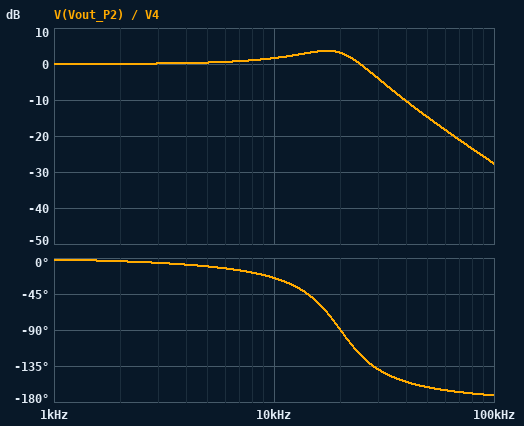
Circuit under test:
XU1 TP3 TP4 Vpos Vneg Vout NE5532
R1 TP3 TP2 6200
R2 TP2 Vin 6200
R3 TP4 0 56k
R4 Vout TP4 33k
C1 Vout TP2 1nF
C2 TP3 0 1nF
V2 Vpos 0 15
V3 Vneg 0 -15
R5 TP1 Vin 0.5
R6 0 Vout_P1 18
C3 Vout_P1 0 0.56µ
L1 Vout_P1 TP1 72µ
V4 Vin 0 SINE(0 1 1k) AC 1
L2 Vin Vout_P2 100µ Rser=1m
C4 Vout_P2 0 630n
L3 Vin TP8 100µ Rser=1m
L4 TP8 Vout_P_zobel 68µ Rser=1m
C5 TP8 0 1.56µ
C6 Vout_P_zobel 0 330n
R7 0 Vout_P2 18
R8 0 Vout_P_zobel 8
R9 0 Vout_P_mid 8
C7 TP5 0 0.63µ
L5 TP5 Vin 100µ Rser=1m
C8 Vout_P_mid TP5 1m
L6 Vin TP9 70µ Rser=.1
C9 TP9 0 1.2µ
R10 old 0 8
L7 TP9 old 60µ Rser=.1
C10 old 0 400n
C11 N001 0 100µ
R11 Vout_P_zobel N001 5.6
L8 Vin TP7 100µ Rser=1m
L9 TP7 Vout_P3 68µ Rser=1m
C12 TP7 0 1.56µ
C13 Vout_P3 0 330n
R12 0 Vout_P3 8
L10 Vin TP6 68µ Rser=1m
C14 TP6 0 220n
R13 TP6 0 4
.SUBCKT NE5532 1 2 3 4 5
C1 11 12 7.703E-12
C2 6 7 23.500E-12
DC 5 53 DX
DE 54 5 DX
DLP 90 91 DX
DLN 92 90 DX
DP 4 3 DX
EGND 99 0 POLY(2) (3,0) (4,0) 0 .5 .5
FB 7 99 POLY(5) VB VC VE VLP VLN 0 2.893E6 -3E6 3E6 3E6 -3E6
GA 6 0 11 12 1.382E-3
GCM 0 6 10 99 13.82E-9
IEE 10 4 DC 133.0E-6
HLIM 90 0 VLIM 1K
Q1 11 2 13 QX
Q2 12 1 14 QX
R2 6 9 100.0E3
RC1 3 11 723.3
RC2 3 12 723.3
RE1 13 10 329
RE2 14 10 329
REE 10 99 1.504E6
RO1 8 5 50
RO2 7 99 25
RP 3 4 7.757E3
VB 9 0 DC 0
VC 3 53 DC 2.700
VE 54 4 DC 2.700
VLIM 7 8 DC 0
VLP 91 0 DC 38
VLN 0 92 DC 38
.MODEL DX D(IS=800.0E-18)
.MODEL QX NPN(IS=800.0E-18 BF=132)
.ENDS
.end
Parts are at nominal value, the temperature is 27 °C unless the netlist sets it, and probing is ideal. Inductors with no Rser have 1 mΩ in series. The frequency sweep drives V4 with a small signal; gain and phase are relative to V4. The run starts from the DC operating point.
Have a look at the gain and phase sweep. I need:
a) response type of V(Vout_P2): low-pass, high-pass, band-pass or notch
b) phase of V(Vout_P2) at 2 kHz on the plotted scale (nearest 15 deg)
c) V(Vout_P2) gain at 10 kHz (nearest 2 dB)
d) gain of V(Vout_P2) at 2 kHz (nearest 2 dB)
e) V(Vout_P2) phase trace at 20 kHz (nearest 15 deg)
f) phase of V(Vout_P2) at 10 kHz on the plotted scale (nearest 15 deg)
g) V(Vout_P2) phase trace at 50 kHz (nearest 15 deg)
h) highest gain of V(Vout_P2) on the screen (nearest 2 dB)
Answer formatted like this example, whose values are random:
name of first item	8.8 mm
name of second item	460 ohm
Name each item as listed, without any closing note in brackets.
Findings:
response type of V(Vout_P2): low-pass, high-pass, band-pass or notch	low-pass
phase of V(Vout_P2) at 2 kHz on the plotted scale	0 deg
V(Vout_P2) gain at 10 kHz	2 dB
gain of V(Vout_P2) at 2 kHz	0 dB
V(Vout_P2) phase trace at 20 kHz	-90 deg
phase of V(Vout_P2) at 10 kHz on the plotted scale	-30 deg
V(Vout_P2) phase trace at 50 kHz	-165 deg
highest gain of V(Vout_P2) on the screen	4 dB
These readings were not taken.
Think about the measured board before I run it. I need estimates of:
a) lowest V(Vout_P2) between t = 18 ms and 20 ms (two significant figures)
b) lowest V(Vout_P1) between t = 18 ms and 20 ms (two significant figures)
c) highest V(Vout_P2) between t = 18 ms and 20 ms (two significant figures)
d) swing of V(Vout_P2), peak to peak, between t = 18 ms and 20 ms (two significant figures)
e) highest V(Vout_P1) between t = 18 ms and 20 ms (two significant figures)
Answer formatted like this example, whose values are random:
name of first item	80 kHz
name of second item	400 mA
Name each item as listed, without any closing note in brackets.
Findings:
lowest V(Vout_P2) between t = 18 ms and 20 ms	-1.0 V
lowest V(Vout_P1) between t = 18 ms and 20 ms	-970 mV
highest V(Vout_P2) between t = 18 ms and 20 ms	1.0 V
swing of V(Vout_P2), peak to peak, between t = 18 ms and 20 ms	2.0 V
highest V(Vout_P1) between t = 18 ms and 20 ms	970 mV
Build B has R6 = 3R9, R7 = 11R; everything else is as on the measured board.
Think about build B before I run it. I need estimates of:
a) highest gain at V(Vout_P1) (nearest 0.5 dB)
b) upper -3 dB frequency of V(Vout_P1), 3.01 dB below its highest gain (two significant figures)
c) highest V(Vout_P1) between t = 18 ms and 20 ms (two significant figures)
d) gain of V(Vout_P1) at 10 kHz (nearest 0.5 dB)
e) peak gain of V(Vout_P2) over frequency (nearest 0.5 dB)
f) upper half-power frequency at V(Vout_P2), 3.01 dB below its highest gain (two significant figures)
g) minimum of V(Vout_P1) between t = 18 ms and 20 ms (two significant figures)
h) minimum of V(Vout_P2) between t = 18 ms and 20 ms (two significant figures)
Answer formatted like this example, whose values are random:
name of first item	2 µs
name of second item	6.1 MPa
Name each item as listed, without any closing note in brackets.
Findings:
highest gain at V(Vout_P1)	-1.0 dB
upper -3 dB frequency of V(Vout_P1), 3.01 dB below its highest gain	11 kHz
highest V(Vout_P1) between t = 18 ms and 20 ms	880 mV
gain of V(Vout_P1) at 10 kHz	-3.5 dB
peak gain of V(Vout_P2) over frequency	0.5 dB
upper half-power frequency at V(Vout_P2), 3.01 dB below its highest gain	23 kHz
minimum of V(Vout_P1) between t = 18 ms and 20 ms	-880 mV
minimum of V(Vout_P2) between t = 18 ms and 20 ms	-1.0 V
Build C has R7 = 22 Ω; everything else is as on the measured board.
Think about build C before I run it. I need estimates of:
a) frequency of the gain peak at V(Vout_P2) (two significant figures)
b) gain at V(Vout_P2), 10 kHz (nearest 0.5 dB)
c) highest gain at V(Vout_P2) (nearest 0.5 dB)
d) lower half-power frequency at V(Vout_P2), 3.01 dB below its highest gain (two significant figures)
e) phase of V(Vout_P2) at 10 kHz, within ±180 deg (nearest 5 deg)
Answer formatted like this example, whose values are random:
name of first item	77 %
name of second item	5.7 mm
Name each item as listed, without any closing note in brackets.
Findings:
frequency of the gain peak at V(Vout_P2)	18 kHz
gain at V(Vout_P2), 10 kHz	2.0 dB
highest gain at V(Vout_P2)	5.0 dB
lower half-power frequency at V(Vout_P2), 3.01 dB below its highest gain	11 kHz
phase of V(Vout_P2) at 10 kHz, within ±180 deg	-20 deg
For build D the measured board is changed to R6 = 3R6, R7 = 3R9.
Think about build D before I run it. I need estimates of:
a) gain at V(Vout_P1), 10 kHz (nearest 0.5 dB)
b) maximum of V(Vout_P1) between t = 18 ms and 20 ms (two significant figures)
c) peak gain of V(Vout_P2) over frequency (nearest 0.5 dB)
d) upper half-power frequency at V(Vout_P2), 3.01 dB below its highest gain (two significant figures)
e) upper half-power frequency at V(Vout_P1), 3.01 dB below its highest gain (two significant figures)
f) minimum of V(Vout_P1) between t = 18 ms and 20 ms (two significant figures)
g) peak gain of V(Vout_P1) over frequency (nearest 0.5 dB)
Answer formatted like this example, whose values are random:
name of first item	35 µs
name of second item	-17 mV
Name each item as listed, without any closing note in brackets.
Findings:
gain at V(Vout_P1), 10 kHz	-4.0 dB
maximum of V(Vout_P1) between t = 18 ms and 20 ms	870 mV
peak gain of V(Vout_P2) over frequency	0 dB
upper half-power frequency at V(Vout_P2), 3.01 dB below its highest gain	6.9 kHz
upper half-power frequency at V(Vout_P1), 3.01 dB below its highest gain	10 kHz
minimum of V(Vout_P1) between t = 18 ms and 20 ms	-870 mV
peak gain of V(Vout_P1) over frequency	-1.0 dB
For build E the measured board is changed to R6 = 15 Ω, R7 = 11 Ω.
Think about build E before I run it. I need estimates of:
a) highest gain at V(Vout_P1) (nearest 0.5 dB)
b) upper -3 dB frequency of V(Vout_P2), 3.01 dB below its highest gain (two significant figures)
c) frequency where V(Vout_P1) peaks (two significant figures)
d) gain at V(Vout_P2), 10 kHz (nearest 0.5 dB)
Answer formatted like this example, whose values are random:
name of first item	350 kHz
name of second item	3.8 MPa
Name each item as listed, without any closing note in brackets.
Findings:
highest gain at V(Vout_P1)	2.5 dB
upper -3 dB frequency of V(Vout_P2), 3.01 dB below its highest gain	23 kHz
frequency where V(Vout_P1) peaks	21 kHz
gain at V(Vout_P2), 10 kHz	0.5 dB
